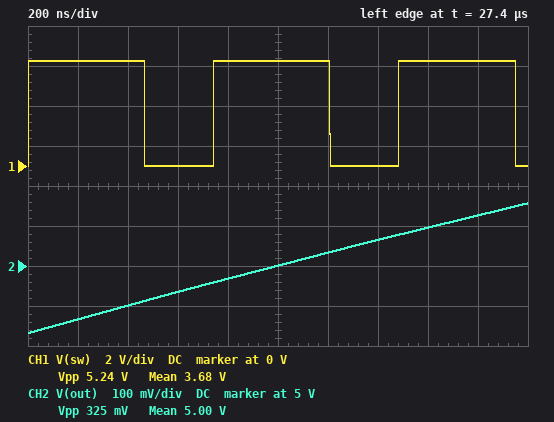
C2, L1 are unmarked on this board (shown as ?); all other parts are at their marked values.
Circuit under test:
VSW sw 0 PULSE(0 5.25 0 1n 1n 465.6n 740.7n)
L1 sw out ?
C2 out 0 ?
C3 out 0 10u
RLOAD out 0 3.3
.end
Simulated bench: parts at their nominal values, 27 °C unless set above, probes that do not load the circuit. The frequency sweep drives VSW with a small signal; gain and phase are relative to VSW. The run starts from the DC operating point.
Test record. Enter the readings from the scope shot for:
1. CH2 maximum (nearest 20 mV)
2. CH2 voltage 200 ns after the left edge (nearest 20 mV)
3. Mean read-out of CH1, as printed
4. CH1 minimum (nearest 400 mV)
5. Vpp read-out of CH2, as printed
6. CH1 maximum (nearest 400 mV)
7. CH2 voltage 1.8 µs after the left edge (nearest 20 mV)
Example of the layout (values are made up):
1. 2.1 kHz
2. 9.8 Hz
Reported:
1. 5.16 V
2. 4.86 V
3. 3.68 V
4. 0 V
5. 325 mV
6. 5.2 V
7. 5.12 V
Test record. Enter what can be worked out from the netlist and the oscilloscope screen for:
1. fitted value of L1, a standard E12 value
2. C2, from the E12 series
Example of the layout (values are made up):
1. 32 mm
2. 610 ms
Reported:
1. 6.8 µH
2. 12 µF
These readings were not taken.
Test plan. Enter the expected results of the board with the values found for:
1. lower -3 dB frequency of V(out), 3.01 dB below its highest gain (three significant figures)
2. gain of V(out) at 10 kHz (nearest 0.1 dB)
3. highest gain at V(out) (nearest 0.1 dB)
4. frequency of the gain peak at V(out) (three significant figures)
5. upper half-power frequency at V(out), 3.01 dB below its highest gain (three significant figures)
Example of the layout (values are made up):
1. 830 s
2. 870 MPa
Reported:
1. 11.8 kHz
2. 7.3 dB
3. 15.5 dB
4. 12.9 kHz
5. 14.0 kHz
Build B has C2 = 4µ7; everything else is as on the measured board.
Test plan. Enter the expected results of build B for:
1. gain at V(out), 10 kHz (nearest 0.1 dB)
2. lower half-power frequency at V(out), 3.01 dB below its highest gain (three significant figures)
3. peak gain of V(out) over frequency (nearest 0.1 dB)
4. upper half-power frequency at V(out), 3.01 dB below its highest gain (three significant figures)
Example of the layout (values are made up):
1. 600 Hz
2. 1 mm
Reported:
1. 4.2 dB
2. 14.0 kHz
3. 13.8 dB
4. 17.3 kHz
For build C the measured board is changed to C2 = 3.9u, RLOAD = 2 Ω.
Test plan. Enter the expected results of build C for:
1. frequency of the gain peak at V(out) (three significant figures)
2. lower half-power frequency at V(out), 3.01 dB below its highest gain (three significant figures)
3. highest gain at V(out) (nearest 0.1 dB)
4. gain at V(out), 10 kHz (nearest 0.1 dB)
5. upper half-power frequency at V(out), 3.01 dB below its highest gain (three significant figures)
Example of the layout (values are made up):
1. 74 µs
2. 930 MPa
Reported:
1. 15.9 kHz
2. 12.6 kHz
3. 9.3 dB
4. 3.6 dB
5. 18.5 kHz
